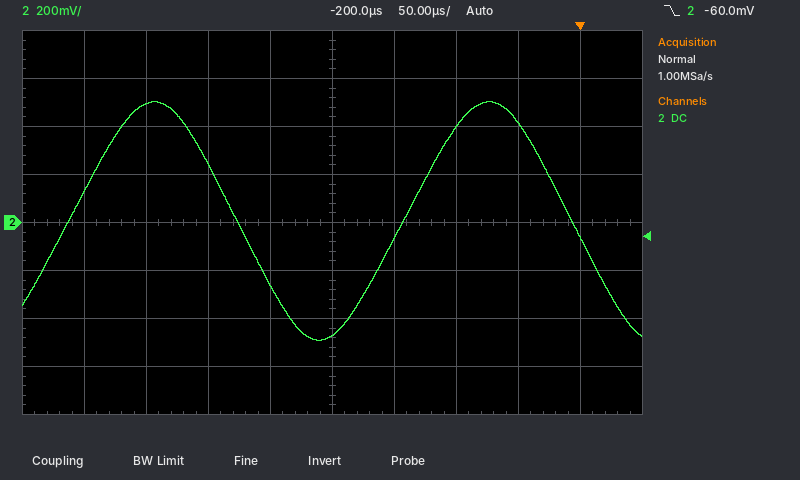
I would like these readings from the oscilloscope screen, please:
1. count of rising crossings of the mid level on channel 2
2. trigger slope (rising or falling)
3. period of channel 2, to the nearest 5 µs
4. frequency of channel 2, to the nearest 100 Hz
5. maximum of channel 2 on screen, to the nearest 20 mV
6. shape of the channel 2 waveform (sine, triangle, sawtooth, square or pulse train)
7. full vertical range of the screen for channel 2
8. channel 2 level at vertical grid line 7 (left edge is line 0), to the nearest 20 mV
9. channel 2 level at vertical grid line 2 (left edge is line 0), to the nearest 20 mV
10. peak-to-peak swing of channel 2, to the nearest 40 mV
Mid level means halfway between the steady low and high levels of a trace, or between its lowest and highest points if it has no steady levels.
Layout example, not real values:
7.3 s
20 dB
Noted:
2
falling
270 µs
3.7 kHz
500 mV
sine
1.6 V
400 mV
500 mV
1.00 V
